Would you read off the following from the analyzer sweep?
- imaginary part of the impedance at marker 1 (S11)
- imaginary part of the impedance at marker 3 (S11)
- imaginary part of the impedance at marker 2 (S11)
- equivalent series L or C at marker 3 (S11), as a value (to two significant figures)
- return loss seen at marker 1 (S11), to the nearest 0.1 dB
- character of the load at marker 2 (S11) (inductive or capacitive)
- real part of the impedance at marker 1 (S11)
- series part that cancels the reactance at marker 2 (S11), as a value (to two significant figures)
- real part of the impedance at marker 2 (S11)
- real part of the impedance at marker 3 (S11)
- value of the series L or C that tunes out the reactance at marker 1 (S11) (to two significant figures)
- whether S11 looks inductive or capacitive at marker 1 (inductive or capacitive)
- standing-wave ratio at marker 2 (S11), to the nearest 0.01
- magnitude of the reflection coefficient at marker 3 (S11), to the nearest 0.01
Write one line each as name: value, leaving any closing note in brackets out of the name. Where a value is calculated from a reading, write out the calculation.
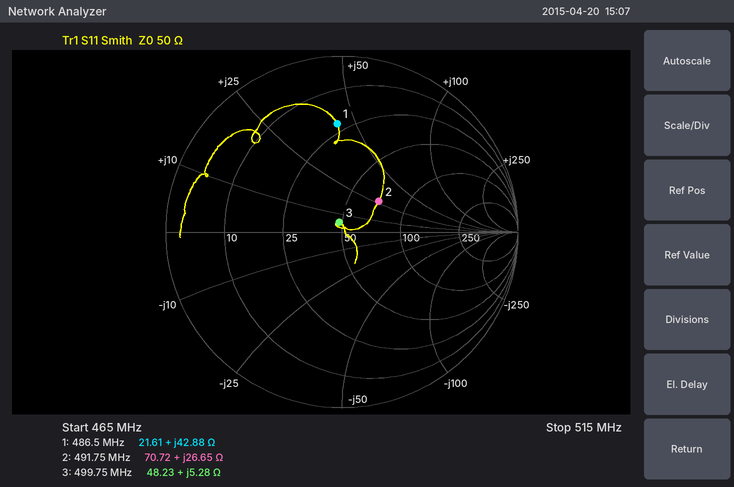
imaginary part of the impedance at marker 1: +42.88 Ω
imaginary part of the impedance at marker 3: +5.28 Ω
imaginary part of the impedance at marker 2: +26.65 Ω
equivalent series L or C at marker 3 (S11), as a value: L = 5.28 Ω/(2π × 499.75 MHz) ≈ 1.7 nH
return loss seen at marker 1 (S11), to the nearest 0.1 dB: 4.2 dB
character of the load at marker 2 (S11): inductive
real part of the impedance at marker 1: 21.61 Ω
series part that cancels the reactance at marker 2 (S11), as a value: C = 1/(2π × 491.75 MHz × 26.65 Ω) ≈ 12 pF
real part of the impedance at marker 2: 70.72 Ω
real part of the impedance at marker 3: 48.23 Ω
value of the series L or C that tunes out the reactance at marker 1 (S11): C = 1/(2π × 486.5 MHz × 42.88 Ω) ≈ 7.6 pF
whether S11 looks inductive or capacitive at marker 1: inductive
standing-wave ratio at marker 2 (S11), to the nearest 0.01: 1.75
magnitude of the reflection coefficient at marker 3 (S11), to the nearest 0.01: 0.06
